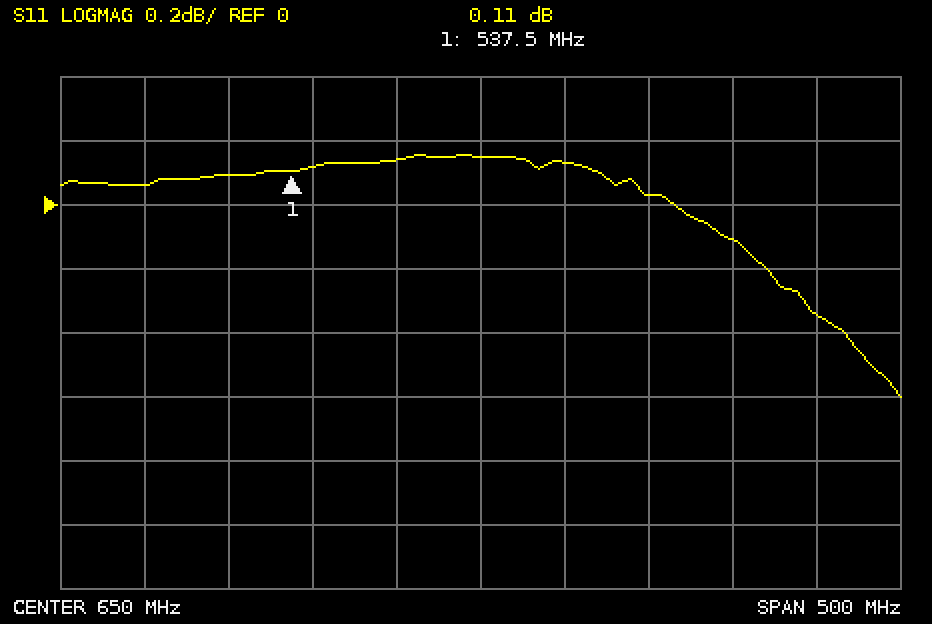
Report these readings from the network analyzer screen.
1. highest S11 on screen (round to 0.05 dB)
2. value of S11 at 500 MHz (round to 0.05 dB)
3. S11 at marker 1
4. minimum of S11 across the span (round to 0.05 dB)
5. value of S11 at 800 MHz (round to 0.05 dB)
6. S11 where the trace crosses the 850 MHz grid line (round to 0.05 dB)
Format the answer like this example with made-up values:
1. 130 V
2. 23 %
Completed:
1. 0.15 dB
2. 0.10 dB
3. 0.11 dB
4. -0.60 dB
5. -0.10 dB
6. -0.35 dB
